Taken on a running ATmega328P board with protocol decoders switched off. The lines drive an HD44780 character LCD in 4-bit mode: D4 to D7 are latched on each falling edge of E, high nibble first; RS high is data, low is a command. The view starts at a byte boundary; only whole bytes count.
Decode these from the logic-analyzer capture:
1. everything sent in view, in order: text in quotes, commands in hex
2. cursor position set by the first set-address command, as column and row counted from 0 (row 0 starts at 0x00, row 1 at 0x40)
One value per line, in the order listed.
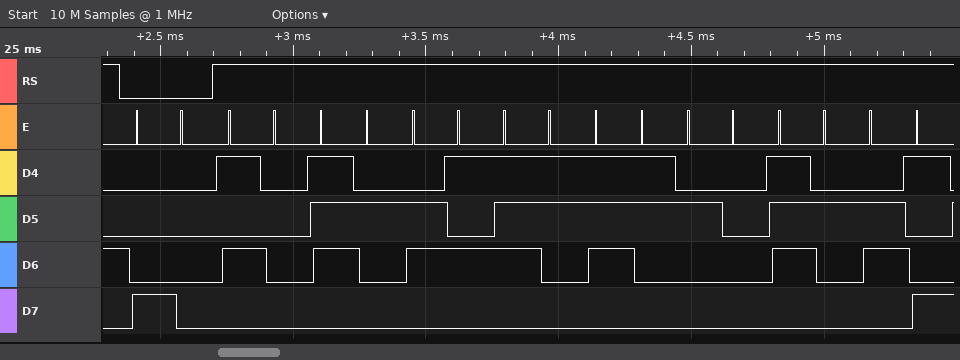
0x80 "Press ri"
column 0, row 0
